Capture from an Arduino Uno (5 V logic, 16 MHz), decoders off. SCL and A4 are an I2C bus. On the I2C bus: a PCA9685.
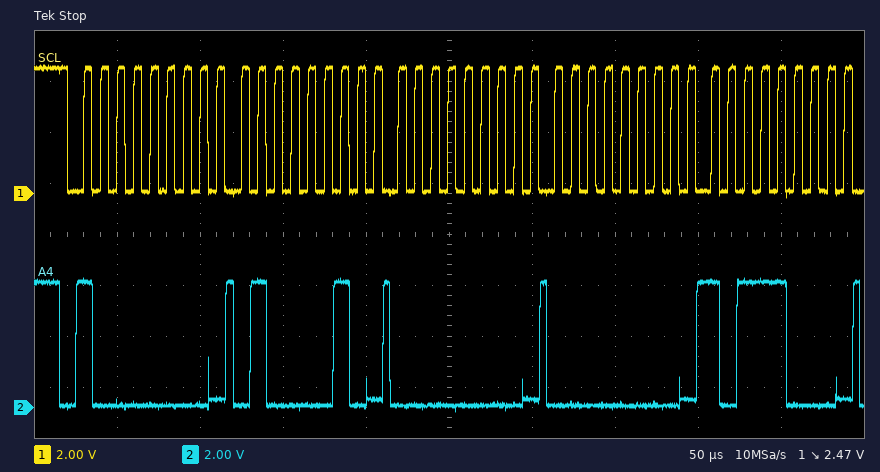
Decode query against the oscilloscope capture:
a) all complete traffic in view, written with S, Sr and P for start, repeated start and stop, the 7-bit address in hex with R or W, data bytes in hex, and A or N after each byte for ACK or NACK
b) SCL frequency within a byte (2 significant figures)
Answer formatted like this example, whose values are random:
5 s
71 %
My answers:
S 40W A 42 A 00 A 00 A B8 A
100 kHz
